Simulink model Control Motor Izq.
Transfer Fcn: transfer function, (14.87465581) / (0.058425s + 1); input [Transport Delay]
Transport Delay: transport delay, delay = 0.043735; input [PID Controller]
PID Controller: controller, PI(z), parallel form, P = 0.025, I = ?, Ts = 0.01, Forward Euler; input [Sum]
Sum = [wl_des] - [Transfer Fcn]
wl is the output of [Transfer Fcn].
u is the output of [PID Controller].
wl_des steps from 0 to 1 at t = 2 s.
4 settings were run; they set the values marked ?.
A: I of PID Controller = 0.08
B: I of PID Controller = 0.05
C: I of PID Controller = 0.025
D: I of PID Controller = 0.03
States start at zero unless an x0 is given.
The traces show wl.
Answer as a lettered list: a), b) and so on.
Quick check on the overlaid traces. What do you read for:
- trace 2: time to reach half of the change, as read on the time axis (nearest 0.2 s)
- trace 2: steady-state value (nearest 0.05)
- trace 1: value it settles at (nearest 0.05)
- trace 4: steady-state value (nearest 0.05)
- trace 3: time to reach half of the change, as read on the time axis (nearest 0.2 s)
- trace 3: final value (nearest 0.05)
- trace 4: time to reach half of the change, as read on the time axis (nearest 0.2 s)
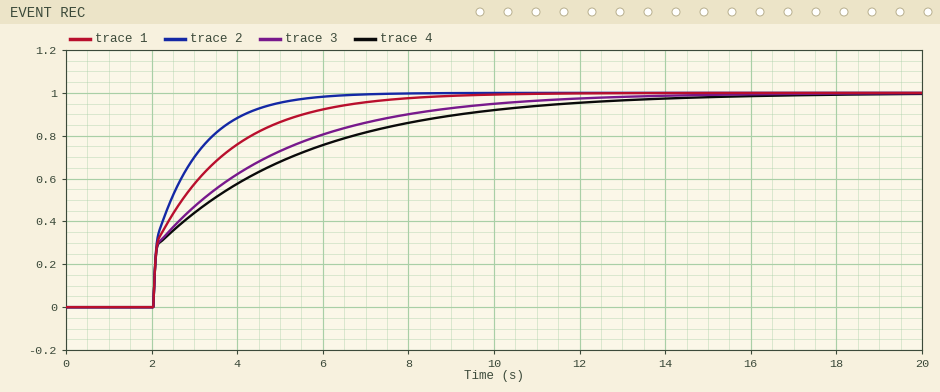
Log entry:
a) 2.4 s
b) 1.00
c) 1.00
d) 1.00
e) 3.2 s
f) 1.00
g) 3.4 s
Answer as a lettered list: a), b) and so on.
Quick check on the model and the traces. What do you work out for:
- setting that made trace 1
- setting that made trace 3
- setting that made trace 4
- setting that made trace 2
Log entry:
a) B
b) D
c) C
d) A
